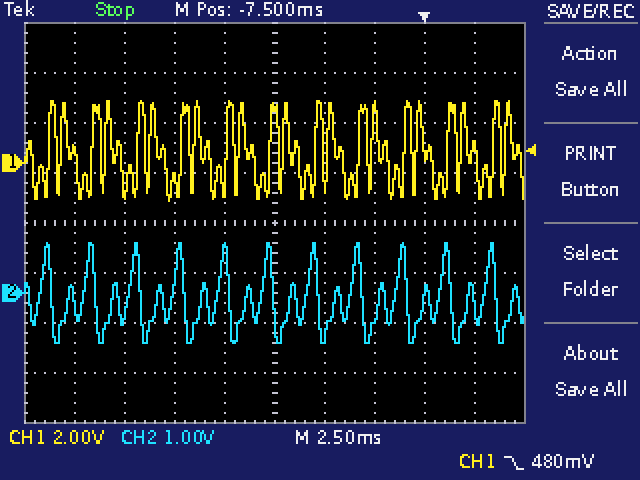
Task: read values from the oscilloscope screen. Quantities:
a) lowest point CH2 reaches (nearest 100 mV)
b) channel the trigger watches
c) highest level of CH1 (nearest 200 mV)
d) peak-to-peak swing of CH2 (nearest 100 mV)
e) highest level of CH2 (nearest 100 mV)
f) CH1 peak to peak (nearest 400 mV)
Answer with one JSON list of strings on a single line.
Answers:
["-1.0 V", "CH1", "2.4 V", "2.0 V", "1.0 V", "4.0 V"]
